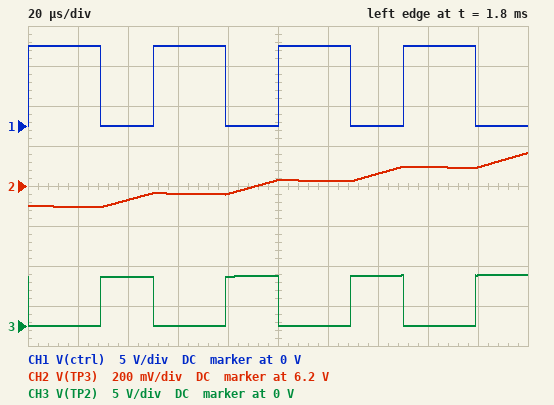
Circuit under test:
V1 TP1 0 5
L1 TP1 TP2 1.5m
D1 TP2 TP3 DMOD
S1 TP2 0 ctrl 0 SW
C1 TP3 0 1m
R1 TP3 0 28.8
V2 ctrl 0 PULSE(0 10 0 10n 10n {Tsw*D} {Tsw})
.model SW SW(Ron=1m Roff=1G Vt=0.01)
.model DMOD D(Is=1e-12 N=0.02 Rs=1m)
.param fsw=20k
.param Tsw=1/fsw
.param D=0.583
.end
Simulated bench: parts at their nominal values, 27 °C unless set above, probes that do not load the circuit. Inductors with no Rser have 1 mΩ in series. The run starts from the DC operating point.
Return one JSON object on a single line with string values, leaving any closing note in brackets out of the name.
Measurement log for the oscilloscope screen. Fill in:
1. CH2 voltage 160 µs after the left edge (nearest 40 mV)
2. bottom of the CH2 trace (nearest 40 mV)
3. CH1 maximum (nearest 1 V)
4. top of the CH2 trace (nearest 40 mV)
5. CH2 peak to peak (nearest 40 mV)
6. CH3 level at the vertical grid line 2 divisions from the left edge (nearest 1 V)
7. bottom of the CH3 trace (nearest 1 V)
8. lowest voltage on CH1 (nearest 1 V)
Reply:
{"CH2 voltage 160 µs after the left edge": "6.28 V", "bottom of the CH2 trace": "6.08 V", "CH1 maximum": "10 V", "top of the CH2 trace": "6.36 V", "CH2 peak to peak": "280 mV", "CH3 level at the vertical grid line 2 divisions from the left edge": "6 V", "bottom of the CH3 trace": "0 V", "lowest voltage on CH1": "0 V"}
